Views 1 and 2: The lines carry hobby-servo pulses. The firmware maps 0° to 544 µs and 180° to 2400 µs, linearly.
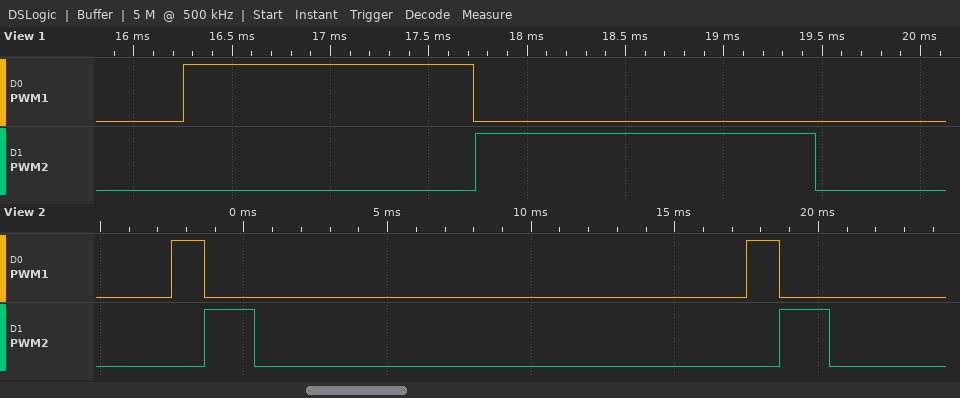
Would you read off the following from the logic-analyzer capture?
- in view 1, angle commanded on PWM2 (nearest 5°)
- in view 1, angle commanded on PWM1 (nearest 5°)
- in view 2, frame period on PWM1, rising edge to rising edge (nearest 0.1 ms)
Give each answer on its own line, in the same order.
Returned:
115°
90°
20.0 ms
